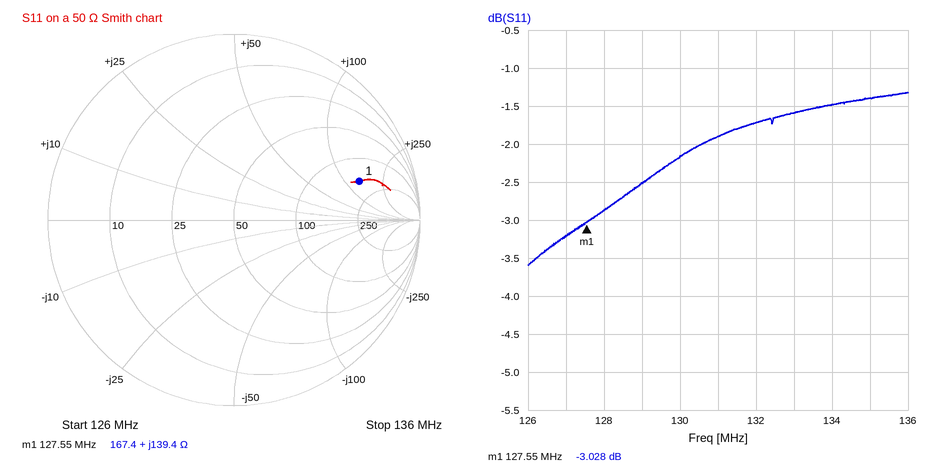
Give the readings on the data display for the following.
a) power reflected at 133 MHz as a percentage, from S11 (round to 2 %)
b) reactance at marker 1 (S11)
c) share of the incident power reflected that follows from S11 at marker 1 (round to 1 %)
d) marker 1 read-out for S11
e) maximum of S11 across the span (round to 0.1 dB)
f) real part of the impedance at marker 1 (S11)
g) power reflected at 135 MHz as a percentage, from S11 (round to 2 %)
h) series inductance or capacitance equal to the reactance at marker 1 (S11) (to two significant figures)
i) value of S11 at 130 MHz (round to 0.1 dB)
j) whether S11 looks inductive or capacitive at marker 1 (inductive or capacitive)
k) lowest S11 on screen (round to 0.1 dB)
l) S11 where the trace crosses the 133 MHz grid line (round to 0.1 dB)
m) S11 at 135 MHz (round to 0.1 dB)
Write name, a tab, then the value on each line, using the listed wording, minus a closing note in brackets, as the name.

power reflected at 133 MHz as a percentage, from S11	70 %
reactance at marker 1	+139.4 Ω
share of the incident power reflected that follows from S11 at marker 1	50 %
marker 1 read-out for S11	-3.028 dB
maximum of S11 across the span	-1.3 dB
real part of the impedance at marker 1	167.4 Ω
power reflected at 135 MHz as a percentage, from S11	72 %
series inductance or capacitance equal to the reactance at marker 1 (S11)	170 nH
value of S11 at 130 MHz	-2.2 dB
whether S11 looks inductive or capacitive at marker 1	inductive
lowest S11 on screen	-3.6 dB
S11 where the trace crosses the 133 MHz grid line	-1.6 dB
S11 at 135 MHz	-1.4 dB
